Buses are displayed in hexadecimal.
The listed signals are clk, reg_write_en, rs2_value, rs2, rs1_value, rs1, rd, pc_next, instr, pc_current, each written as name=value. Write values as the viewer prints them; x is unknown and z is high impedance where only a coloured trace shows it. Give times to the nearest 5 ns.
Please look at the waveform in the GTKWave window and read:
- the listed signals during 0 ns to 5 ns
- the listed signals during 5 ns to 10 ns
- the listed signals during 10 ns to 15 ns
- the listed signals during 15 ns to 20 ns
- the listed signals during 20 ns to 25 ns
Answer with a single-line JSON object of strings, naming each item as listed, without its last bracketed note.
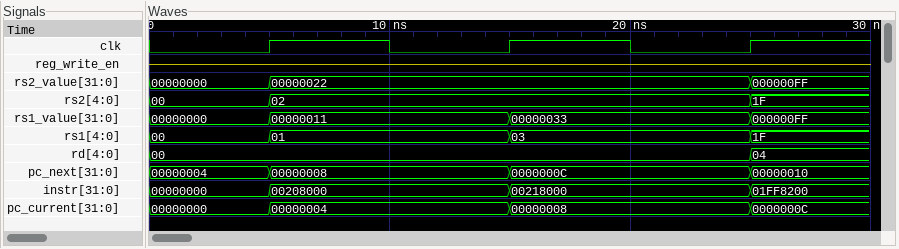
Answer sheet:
{"the listed signals during 0 ns to 5 ns": "clk=0, reg_write_en=z, rs2_value=00000000, rs2=00, rs1_value=00000000, rs1=00, rd=00, pc_next=00000004, instr=00000000, pc_current=00000000", "the listed signals during 5 ns to 10 ns": "clk=1, reg_write_en=z, rs2_value=00000022, rs2=02, rs1_value=00000011, rs1=01, rd=00, pc_next=00000008, instr=00208000, pc_current=00000004", "the listed signals during 10 ns to 15 ns": "clk=0, reg_write_en=z, rs2_value=00000022, rs2=02, rs1_value=00000011, rs1=01, rd=00, pc_next=00000008, instr=00208000, pc_current=00000004", "the listed signals during 15 ns to 20 ns": "clk=1, reg_write_en=z, rs2_value=00000022, rs2=02, rs1_value=00000033, rs1=03, rd=00, pc_next=0000000C, instr=00218000, pc_current=00000008", "the listed signals during 20 ns to 25 ns": "clk=0, reg_write_en=z, rs2_value=00000022, rs2=02, rs1_value=00000033, rs1=03, rd=00, pc_next=0000000C, instr=00218000, pc_current=00000008"}
